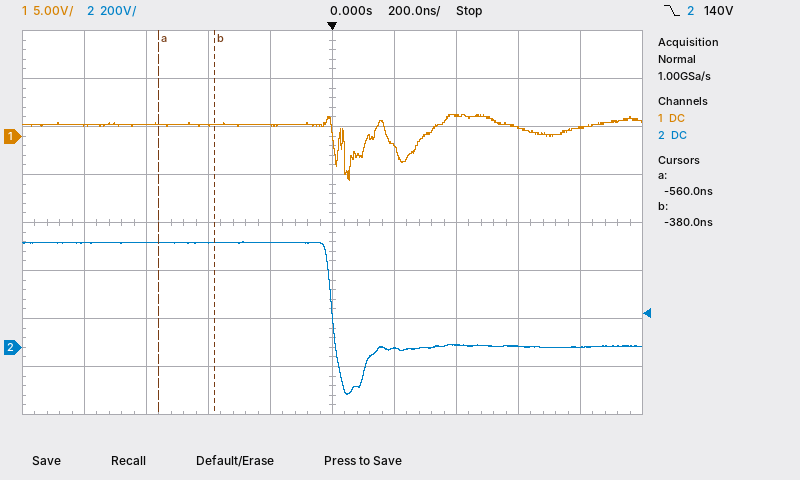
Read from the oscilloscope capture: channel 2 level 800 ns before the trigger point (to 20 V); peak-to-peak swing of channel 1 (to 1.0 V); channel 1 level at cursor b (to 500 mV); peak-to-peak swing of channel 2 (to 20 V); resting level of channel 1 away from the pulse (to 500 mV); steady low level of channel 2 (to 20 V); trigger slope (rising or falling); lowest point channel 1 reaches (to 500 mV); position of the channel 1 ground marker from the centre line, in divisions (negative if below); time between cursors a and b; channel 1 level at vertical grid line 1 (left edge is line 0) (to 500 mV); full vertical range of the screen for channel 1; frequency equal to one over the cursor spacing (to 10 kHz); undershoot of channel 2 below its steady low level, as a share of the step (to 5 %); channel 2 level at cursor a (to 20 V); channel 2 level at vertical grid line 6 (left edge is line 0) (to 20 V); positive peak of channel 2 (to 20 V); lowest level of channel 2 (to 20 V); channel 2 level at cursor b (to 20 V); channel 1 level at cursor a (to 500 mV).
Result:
440 V
7.0 V
1.0 V
640 V
1.0 V
0 V
falling
-4.5 V
+1.8 div
180 ns
1.0 V
40 V
5.56 MHz
45 %
440 V
0 V
440 V
-200 V
440 V
1.5 V
